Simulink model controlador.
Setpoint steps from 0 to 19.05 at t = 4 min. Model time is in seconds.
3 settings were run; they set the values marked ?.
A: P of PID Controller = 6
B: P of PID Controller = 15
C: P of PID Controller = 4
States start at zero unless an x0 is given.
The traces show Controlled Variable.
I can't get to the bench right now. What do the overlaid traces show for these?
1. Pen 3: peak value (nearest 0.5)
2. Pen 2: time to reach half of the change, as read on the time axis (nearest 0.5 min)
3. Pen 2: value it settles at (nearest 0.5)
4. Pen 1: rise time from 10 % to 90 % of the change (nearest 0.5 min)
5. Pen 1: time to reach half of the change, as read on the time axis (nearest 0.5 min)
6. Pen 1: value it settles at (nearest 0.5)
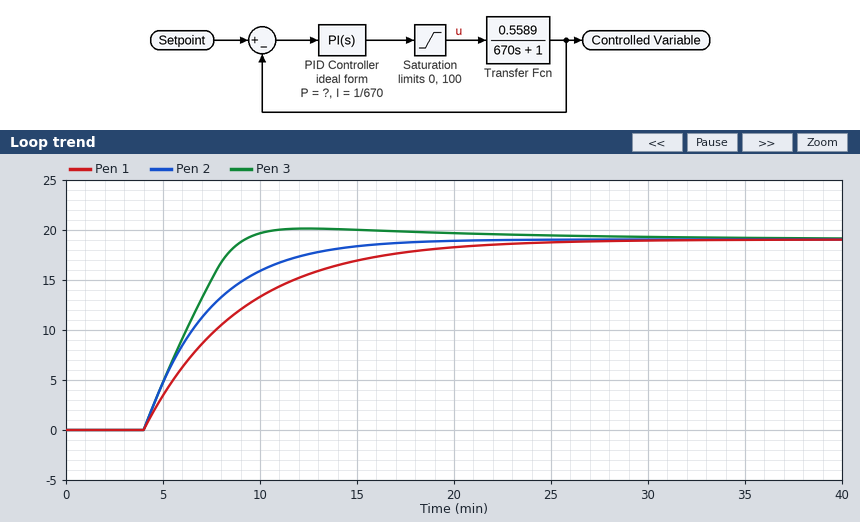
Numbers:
20.0
6.5 min
19.0
11.0 min
7.5 min
19.0
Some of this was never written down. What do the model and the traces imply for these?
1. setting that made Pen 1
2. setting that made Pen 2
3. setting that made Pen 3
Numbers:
C
A
B
